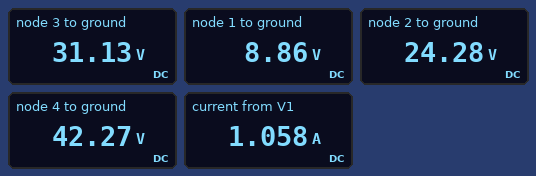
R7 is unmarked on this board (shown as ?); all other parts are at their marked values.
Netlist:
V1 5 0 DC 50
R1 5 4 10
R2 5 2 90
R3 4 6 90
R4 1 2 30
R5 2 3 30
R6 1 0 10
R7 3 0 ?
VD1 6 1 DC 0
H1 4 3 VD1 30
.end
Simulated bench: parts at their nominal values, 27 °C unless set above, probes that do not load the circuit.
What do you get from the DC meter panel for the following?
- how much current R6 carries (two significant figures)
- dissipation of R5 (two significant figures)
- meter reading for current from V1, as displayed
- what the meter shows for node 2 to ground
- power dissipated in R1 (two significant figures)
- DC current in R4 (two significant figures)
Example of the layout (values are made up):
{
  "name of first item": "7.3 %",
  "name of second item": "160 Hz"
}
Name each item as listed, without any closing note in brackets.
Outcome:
{
  "how much current R6 carries": "890 mA",
  "dissipation of R5": "1.6 W",
  "meter reading for current from V1, as displayed": "1.058 A",
  "what the meter shows for node 2 to ground": "24.28 V",
  "power dissipated in R1": "6.0 W",
  "DC current in R4": "510 mA"
}
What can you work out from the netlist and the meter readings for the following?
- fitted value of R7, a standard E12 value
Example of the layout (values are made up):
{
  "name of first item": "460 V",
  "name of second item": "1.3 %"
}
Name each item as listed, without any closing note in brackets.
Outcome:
{
  "fitted value of R7, a standard E12 value": "180 Ω"
}
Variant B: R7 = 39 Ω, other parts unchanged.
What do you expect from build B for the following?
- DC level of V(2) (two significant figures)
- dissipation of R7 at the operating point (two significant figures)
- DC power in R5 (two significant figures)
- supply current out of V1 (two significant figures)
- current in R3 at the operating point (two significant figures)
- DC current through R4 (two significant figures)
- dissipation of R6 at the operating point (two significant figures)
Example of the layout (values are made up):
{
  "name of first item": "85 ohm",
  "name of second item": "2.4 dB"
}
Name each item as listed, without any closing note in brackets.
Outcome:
{
  "DC level of V(2)": "23 V",
  "dissipation of R7 at the operating point": "20 W",
  "DC power in R5": "940 mW",
  "supply current out of V1": "1.5 A",
  "current in R3 at the operating point": "330 mA",
  "DC current through R4": "480 mA",
  "dissipation of R6 at the operating point": "6.6 W"
}
